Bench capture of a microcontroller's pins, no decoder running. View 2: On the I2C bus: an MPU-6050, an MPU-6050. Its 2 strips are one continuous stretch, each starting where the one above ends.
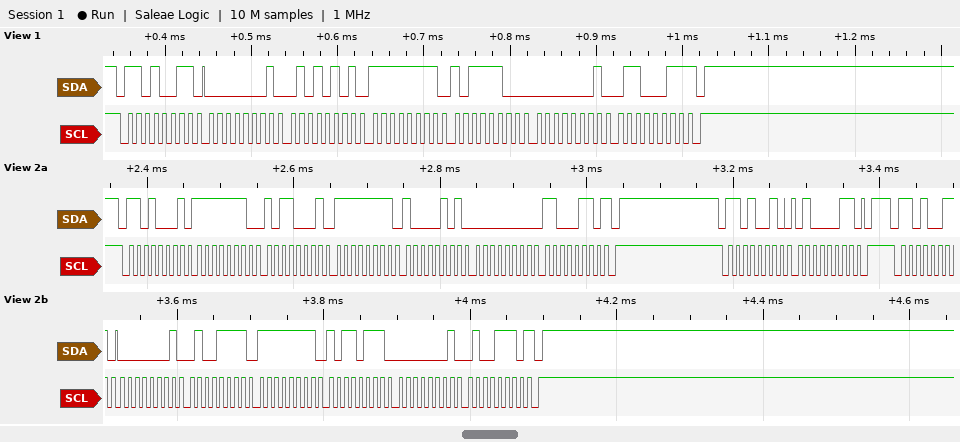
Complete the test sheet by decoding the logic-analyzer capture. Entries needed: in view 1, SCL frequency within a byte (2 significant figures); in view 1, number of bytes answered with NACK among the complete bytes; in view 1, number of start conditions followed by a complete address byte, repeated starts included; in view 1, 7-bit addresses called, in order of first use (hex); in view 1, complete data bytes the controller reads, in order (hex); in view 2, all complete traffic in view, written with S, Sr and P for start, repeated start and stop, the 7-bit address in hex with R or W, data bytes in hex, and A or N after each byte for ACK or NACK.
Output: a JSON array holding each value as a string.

["100 kHz", "1", "1", "0x69", "01 55 FF BC 01 63", "S 68R A FE A B1 A FF A 85 A 00 A C6 N P S 69W A 43 A P S 69R A 01 A 4F A FF A B7 A 01 A 4E N P"]
